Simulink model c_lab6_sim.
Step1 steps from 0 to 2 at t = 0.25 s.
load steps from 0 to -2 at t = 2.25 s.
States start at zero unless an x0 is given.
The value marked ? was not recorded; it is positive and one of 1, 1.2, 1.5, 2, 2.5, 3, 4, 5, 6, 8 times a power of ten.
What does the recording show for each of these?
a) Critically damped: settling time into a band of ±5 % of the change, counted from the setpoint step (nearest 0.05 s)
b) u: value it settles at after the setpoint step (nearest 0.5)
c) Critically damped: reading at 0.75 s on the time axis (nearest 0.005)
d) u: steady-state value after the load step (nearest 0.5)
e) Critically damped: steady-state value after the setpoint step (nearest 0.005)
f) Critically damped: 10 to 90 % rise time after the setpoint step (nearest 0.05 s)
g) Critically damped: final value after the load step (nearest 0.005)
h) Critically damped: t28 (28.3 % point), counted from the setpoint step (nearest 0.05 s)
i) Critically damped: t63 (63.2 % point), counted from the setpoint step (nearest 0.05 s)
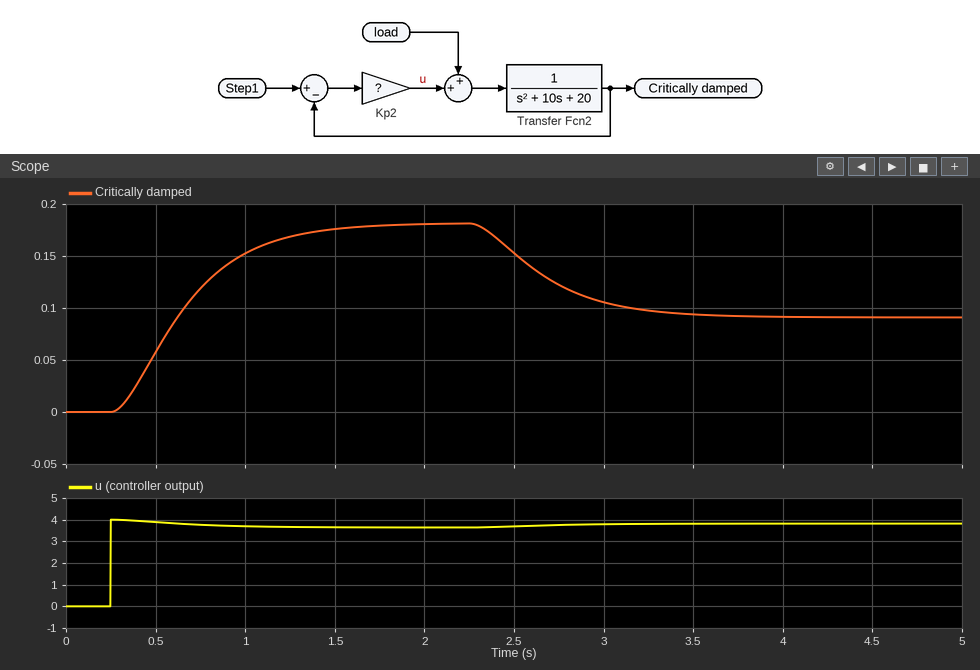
1.10 s
3.5
0.120
4.0
0.180
0.80 s
0.090
0.25 s
0.50 s
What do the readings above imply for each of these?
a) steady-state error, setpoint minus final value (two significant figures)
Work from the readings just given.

1.8
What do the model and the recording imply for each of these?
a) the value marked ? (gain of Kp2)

2
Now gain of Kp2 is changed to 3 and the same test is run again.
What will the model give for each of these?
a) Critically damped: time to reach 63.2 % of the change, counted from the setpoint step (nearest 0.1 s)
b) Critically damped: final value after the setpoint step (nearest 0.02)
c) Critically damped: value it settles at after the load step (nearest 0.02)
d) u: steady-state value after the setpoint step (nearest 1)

0.5 s
0.26
0.18
5
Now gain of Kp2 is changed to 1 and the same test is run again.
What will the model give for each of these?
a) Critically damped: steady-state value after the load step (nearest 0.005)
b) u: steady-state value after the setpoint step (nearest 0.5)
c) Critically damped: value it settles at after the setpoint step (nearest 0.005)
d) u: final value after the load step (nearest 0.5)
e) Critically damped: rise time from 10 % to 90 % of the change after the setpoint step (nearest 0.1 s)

0.000
2.0
0.095
2.0
0.8 s
